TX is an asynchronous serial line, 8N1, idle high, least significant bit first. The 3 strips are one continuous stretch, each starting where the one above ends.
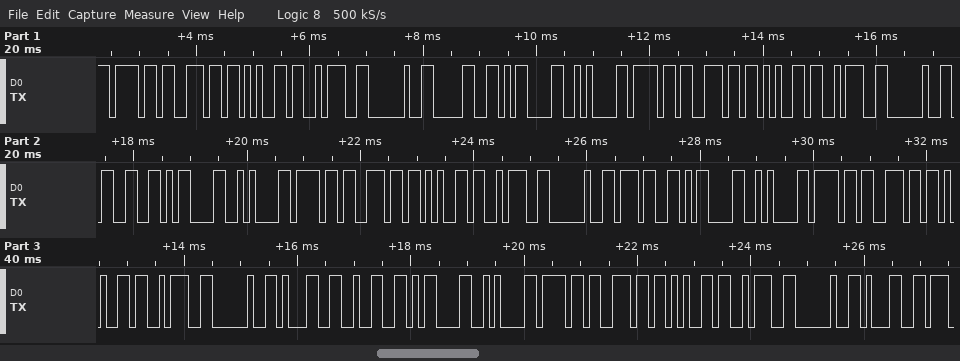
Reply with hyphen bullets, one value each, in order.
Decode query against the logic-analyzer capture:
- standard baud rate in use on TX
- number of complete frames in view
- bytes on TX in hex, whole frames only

- 9600 baud
- 39
- 0x6F 0x6E 0x65 0x3A 0x20 0x30 0x0D 0x0A 0x6F 0x6E 0x65 0x3A 0x20 0x33 0x0D 0x0A 0x6F 0x6E 0x65 0x3A 0x20 0x37 0x0D 0x0A 0x6F 0x6E 0x65 0x3A 0x20 0x31 0x32 0x0D 0x0A 0x6F 0x6E 0x65 0x3A 0x20 0x31
